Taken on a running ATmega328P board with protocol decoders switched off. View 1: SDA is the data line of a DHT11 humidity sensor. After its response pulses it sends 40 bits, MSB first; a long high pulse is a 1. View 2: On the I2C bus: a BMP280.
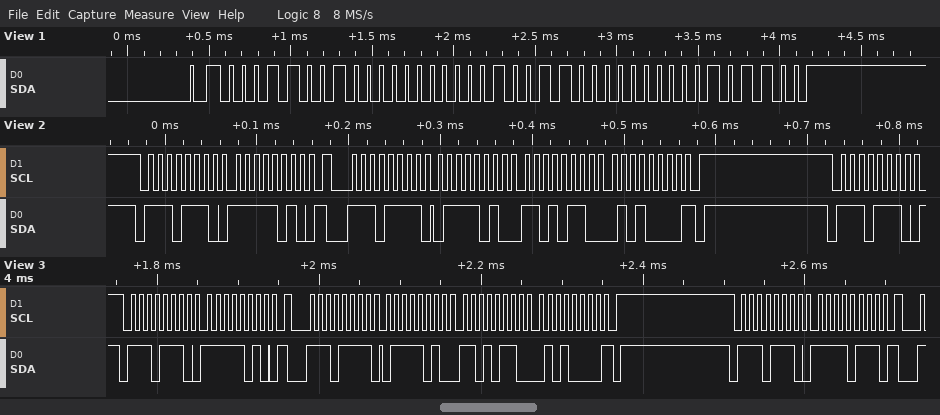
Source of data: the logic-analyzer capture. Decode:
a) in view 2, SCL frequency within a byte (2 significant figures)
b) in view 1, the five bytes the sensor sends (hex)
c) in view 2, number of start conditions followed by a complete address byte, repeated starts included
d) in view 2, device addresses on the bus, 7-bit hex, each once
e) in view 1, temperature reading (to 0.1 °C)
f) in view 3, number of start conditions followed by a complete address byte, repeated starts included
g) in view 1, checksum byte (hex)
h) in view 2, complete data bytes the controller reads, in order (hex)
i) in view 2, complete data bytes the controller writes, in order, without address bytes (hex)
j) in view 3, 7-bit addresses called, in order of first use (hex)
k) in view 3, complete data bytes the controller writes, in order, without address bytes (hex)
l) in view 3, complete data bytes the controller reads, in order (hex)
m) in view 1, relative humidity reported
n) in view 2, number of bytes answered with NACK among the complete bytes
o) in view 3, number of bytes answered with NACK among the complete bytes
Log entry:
100 kHz
19 00 13 00 2C
3
0x77
19.0 °C
3
0x2C
7A D6 50
FA
0x77
FA F7
7A D6 50
25 %
1
1
